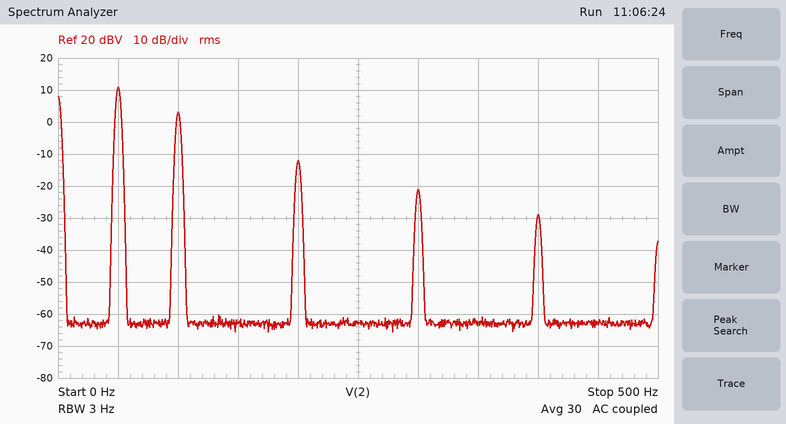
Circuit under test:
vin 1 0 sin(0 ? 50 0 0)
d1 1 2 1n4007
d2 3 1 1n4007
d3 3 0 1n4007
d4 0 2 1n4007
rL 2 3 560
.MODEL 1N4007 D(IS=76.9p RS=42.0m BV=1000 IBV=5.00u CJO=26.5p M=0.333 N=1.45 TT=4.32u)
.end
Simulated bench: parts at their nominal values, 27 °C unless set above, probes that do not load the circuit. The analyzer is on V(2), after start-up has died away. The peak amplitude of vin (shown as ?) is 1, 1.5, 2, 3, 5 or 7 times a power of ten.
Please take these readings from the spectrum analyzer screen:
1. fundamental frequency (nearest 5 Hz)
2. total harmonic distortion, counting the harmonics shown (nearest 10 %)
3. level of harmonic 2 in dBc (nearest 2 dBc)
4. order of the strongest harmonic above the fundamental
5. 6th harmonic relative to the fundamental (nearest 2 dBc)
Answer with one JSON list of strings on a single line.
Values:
["50 Hz", "40 %", "-8 dBc", "2", "-32 dBc"]
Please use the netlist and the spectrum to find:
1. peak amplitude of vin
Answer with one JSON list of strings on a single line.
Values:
["10 V"]
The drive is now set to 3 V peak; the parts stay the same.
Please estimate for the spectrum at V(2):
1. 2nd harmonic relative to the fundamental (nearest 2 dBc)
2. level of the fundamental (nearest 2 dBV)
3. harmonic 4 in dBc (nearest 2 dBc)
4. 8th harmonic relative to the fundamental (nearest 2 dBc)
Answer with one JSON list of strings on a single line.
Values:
["-10 dBc", "0 dBV", "-50 dBc", "-38 dBc"]
